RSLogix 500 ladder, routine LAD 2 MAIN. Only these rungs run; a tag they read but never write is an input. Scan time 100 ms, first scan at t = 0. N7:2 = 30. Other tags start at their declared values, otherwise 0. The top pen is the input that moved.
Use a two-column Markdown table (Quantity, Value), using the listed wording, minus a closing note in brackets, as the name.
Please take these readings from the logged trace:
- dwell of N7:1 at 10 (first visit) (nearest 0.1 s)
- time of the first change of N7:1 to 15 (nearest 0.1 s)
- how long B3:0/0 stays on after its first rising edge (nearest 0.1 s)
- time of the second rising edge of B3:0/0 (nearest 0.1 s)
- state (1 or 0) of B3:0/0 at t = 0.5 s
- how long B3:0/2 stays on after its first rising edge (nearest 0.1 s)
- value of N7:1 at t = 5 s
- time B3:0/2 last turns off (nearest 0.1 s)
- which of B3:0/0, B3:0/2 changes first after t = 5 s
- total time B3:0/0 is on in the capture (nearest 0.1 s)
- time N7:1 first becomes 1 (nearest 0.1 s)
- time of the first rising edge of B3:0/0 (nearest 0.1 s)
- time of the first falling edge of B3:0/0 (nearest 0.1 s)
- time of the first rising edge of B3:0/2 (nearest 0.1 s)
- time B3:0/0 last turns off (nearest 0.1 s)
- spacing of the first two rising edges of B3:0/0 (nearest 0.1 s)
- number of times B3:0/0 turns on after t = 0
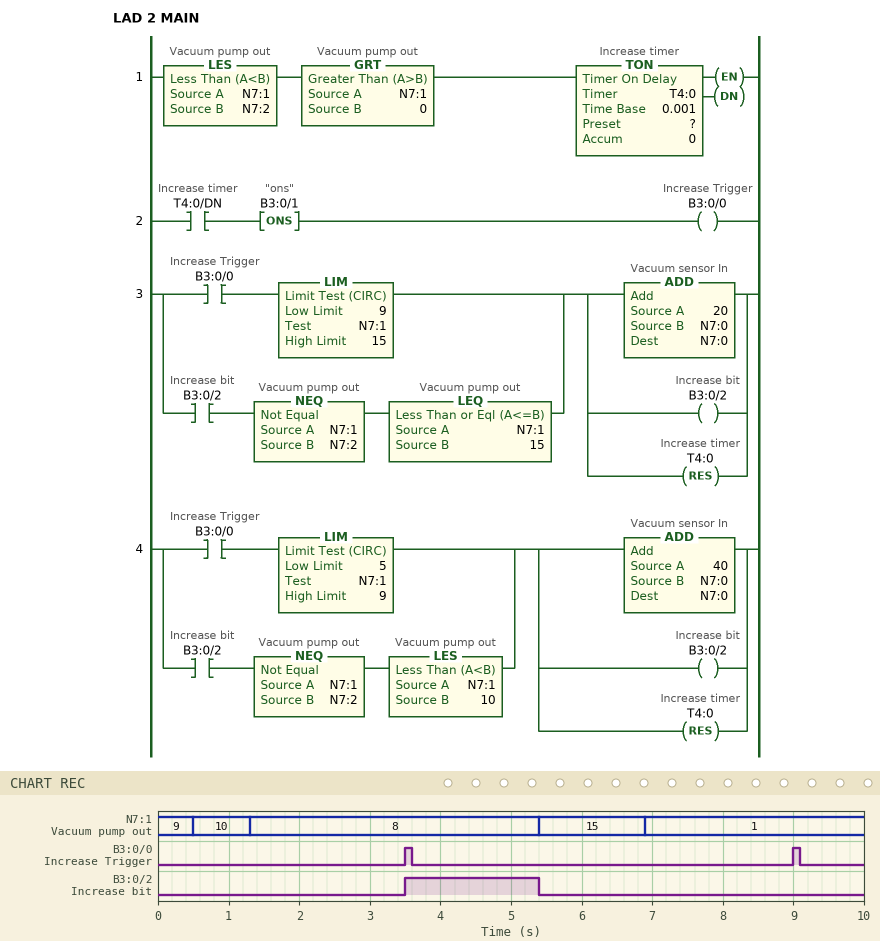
| Quantity | Value |
|---|---|
| dwell of N7:1 at 10 (first visit) | 0.8 s |
| time of the first change of N7:1 to 15 | 5.4 s |
| how long B3:0/0 stays on after its first rising edge | 0.1 s |
| time of the second rising edge of B3:0/0 | 9.0 s |
| state (1 or 0) of B3:0/0 at t = 0.5 s | 0 |
| how long B3:0/2 stays on after its first rising edge | 1.9 s |
| value of N7:1 at t = 5 s | 8 |
| time B3:0/2 last turns off | 5.4 s |
| which of B3:0/0, B3:0/2 changes first after t = 5 s | B3:0/2 |
| total time B3:0/0 is on in the capture | 0.2 s |
| time N7:1 first becomes 1 | 6.9 s |
| time of the first rising edge of B3:0/0 | 3.5 s |
| time of the first falling edge of B3:0/0 | 3.6 s |
| time of the first rising edge of B3:0/2 | 3.5 s |
| time B3:0/0 last turns off | 9.1 s |
| spacing of the first two rising edges of B3:0/0 | 5.5 s |
| number of times B3:0/0 turns on after t = 0 | 2 |
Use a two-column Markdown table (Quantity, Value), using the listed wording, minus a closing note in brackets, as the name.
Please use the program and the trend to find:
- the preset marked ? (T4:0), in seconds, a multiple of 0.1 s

| Quantity | Value |
|---|---|
| the preset marked ? (T4:0), in seconds, a multiple of 0.1 s | 3.5 s |
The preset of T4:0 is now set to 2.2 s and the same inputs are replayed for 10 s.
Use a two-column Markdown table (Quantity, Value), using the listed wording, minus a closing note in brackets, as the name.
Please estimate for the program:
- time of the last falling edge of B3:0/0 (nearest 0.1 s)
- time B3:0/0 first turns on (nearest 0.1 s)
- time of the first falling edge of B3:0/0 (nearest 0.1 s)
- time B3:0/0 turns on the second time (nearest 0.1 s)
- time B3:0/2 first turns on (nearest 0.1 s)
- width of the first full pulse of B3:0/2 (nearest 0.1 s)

| Quantity | Value |
|---|---|
| time of the last falling edge of B3:0/0 | 7.8 s |
| time B3:0/0 first turns on | 2.2 s |
| time of the first falling edge of B3:0/0 | 2.3 s |
| time B3:0/0 turns on the second time | 7.7 s |
| time B3:0/2 first turns on | 2.2 s |
| width of the first full pulse of B3:0/2 | 3.2 s |
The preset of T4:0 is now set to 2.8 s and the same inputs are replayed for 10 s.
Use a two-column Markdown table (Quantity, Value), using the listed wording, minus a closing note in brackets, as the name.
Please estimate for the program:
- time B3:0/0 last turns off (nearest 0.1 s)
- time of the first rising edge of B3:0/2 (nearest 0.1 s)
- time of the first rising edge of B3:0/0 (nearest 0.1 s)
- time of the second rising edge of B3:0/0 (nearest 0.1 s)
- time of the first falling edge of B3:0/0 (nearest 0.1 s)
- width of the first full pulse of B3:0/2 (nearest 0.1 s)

| Quantity | Value |
|---|---|
| time B3:0/0 last turns off | 8.4 s |
| time of the first rising edge of B3:0/2 | 2.8 s |
| time of the first rising edge of B3:0/0 | 2.8 s |
| time of the second rising edge of B3:0/0 | 8.3 s |
| time of the first falling edge of B3:0/0 | 2.9 s |
| width of the first full pulse of B3:0/2 | 2.6 s |
